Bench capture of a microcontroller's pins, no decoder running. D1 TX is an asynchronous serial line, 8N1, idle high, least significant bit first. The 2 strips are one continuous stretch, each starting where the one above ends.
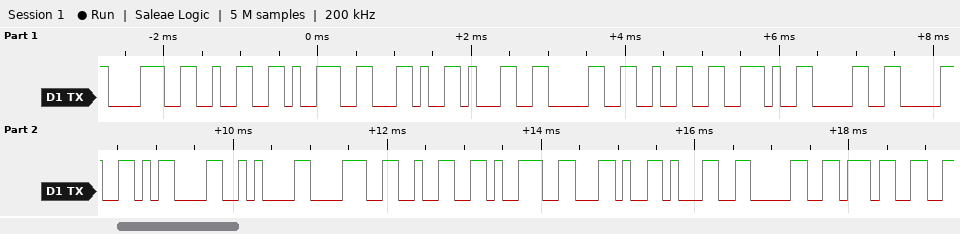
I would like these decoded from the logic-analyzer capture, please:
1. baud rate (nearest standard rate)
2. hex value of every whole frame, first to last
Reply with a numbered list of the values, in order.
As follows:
1. 9600 baud
2. 0x38 0x32 0x39 0x2C 0x31 0x30 0x32 0x2E 0x30 0x30 0x0D 0x0A 0x38 0x32 0x39 0x2C 0x31 0x30 0x37
